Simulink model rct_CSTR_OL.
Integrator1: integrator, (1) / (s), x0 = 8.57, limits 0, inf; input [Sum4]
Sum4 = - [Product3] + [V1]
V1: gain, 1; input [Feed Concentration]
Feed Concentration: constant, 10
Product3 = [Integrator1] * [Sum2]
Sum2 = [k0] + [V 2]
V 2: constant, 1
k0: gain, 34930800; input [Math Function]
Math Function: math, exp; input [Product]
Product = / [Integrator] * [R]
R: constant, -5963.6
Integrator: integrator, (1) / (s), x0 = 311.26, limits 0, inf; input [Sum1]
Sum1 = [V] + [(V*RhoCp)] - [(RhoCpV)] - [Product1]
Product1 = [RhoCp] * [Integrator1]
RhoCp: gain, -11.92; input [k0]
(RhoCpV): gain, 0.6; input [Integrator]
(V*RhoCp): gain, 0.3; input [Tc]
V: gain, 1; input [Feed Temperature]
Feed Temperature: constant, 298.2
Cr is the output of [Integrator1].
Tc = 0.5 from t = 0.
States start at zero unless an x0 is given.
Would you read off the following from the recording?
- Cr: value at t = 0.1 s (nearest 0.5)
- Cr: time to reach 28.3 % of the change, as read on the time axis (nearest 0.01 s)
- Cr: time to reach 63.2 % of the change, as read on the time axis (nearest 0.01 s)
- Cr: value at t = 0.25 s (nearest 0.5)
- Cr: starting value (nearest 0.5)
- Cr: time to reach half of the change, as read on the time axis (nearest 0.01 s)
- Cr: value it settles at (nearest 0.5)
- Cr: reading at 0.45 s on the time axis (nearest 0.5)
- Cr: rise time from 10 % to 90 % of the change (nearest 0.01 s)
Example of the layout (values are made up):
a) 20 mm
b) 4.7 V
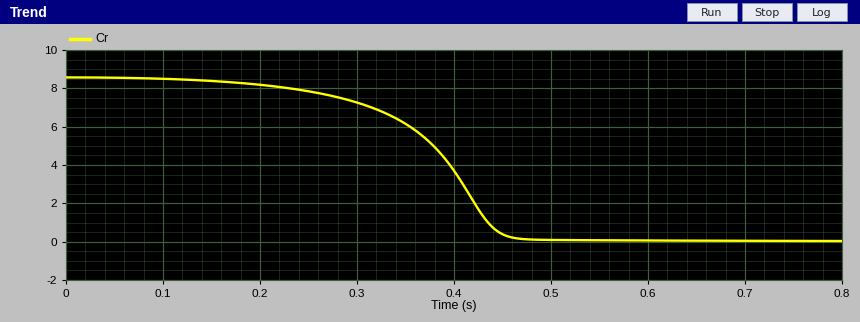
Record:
a) 8.5
b) 0.35 s
c) 0.41 s
d) 8.0
e) 8.5
f) 0.39 s
g) 0.0
h) 0.5
i) 0.17 s
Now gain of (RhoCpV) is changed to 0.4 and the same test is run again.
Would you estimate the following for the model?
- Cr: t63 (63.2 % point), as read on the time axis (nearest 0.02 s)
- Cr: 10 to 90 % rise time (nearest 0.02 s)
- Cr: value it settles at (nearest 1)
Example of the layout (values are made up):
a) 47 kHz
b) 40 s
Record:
a) 0.30 s
b) 0.12 s
c) 0
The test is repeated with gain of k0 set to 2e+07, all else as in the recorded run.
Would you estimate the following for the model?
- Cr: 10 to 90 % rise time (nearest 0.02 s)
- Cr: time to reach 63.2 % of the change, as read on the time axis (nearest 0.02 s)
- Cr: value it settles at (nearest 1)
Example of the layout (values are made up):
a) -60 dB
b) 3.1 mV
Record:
a) 0.20 s
b) 0.52 s
c) 0
